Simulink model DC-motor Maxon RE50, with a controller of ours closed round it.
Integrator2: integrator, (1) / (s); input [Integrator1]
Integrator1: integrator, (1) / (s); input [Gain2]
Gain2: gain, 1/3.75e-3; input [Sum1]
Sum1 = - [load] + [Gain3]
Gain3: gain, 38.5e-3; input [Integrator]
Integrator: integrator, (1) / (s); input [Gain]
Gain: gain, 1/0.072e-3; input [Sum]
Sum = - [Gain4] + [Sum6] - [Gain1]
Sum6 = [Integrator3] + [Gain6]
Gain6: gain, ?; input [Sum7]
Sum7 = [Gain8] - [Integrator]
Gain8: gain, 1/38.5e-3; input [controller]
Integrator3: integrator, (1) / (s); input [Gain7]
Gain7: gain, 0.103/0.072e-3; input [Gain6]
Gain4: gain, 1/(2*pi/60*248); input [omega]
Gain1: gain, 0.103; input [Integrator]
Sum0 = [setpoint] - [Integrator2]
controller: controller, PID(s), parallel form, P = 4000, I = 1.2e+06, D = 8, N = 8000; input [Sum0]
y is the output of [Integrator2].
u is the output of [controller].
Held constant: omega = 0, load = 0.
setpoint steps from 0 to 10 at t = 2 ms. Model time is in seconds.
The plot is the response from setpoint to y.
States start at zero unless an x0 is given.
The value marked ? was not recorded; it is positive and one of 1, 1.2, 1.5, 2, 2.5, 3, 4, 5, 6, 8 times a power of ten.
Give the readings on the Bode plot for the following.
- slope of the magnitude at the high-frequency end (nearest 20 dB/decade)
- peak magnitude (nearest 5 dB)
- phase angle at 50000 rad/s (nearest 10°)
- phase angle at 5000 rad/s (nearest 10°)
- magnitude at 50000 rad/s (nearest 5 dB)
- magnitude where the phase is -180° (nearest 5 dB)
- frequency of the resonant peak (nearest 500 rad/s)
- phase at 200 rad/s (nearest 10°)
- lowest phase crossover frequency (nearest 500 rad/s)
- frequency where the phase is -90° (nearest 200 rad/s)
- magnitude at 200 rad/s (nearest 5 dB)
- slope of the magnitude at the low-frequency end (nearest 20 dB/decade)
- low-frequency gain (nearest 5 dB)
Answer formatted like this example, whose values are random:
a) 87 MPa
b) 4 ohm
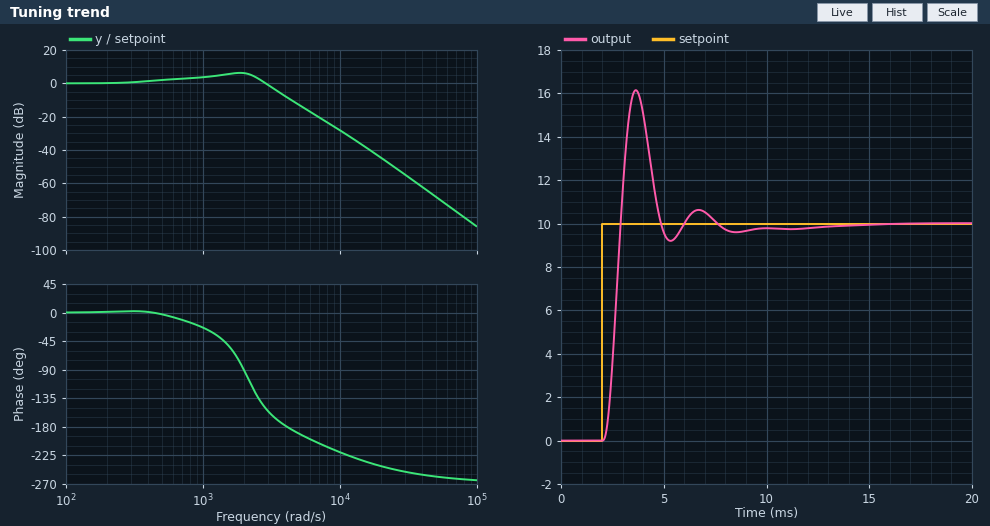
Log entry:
a) -60 dB/decade
b) 5 dB
c) -260°
d) -190°
e) -70 dB
f) -10 dB
g) 2000 rad/s
h) 0°
i) 4000 rad/s
j) 2000 rad/s
k) 0 dB
l) 0 dB/decade
m) 0 dB
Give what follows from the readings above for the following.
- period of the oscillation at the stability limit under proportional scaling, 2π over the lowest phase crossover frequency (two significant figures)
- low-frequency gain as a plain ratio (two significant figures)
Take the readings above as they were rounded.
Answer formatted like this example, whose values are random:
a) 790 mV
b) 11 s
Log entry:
a) 0.0016 s
b) 1.0
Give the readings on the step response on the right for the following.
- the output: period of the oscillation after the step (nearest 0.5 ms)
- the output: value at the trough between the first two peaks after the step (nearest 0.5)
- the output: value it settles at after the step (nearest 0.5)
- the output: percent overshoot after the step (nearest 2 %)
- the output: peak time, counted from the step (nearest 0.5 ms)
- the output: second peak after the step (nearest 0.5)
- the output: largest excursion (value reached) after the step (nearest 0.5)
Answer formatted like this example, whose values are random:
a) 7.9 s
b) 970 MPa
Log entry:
a) 3.0 ms
b) 9.0
c) 10.0
d) 62 %
e) 1.5 ms
f) 10.5
g) 16.0
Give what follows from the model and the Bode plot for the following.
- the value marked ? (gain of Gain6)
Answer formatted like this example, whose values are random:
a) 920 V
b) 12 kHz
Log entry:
a) 0.2
